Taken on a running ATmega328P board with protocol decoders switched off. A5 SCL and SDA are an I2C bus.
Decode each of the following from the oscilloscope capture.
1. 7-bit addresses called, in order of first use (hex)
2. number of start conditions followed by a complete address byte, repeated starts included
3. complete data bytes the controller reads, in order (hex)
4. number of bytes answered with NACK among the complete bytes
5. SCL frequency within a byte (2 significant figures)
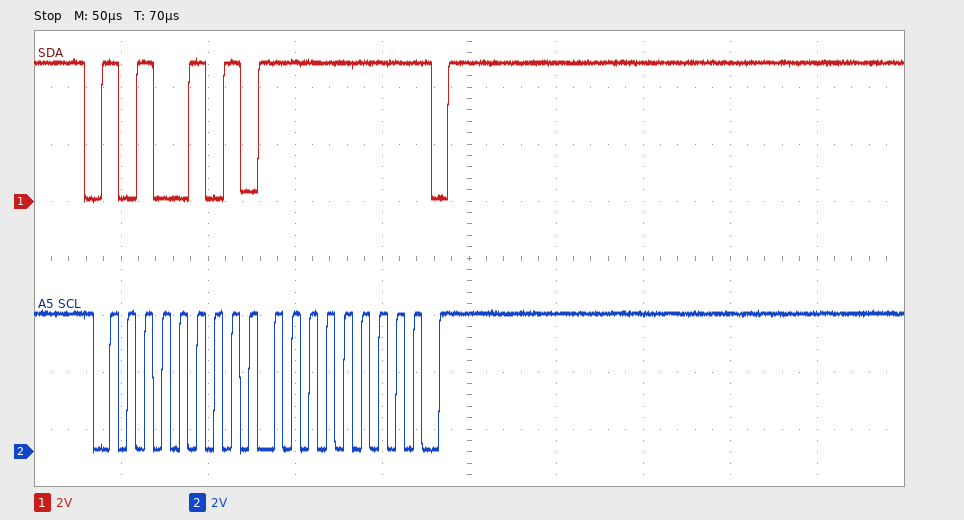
0x52
1
FF
1
100 kHz
